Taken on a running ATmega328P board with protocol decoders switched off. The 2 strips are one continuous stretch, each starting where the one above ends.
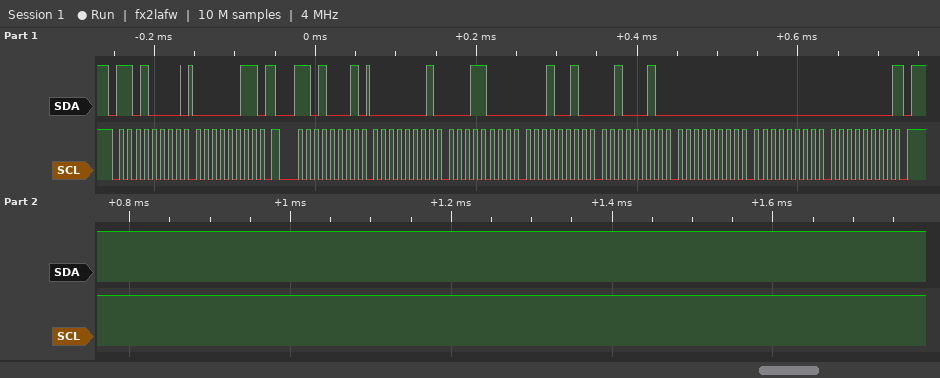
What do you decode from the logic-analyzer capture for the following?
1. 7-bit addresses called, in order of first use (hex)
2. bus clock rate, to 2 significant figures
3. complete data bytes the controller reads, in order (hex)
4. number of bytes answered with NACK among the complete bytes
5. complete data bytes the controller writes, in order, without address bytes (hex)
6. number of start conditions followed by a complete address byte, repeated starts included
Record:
0x68
100 kHz
01 18 12 22 00 00 00
1
03
2
